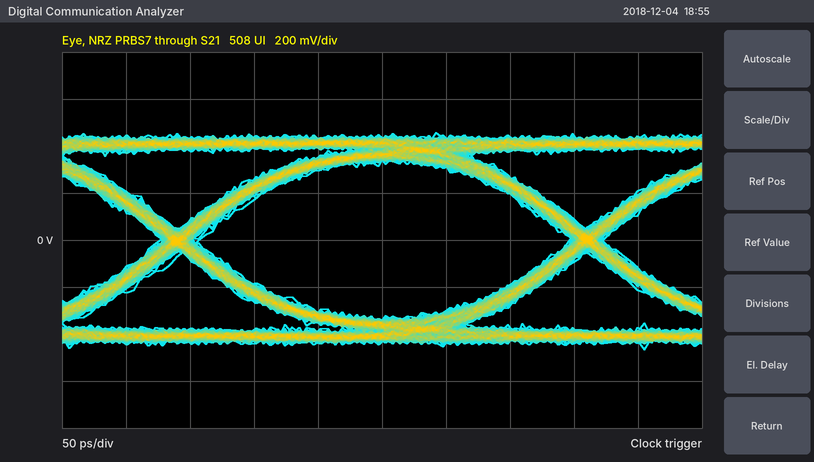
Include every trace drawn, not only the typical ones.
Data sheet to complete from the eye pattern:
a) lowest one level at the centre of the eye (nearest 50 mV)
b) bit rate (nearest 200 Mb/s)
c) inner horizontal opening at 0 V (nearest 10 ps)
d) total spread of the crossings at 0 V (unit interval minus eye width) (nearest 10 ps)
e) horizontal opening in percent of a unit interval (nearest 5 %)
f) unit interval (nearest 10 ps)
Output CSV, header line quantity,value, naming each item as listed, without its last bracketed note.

quantity,value
lowest one level at the centre of the eye,350 mV
bit rate,3.2 Gb/s
inner horizontal opening at 0 V,290 ps
total spread of the crossings at 0 V (unit interval minus eye width),30 ps
horizontal opening in percent of a unit interval,90 %
unit interval,320 ps
